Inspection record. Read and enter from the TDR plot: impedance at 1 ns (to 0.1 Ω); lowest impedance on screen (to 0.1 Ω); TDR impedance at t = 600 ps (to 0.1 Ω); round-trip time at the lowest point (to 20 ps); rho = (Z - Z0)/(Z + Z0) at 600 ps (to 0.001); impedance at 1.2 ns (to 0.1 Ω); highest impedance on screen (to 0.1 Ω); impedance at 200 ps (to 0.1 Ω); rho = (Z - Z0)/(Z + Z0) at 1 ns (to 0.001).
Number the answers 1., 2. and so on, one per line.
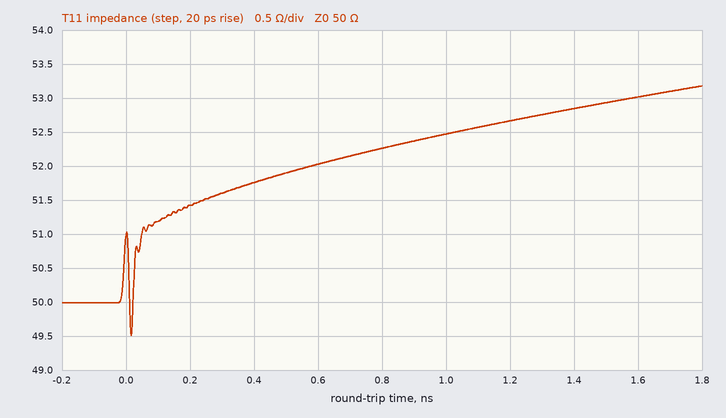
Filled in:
1. 52.5 Ω
2. 49.5 Ω
3. 52.0 Ω
4. 20 ps
5. +0.020
6. 52.7 Ω
7. 53.2 Ω
8. 51.4 Ω
9. +0.024
